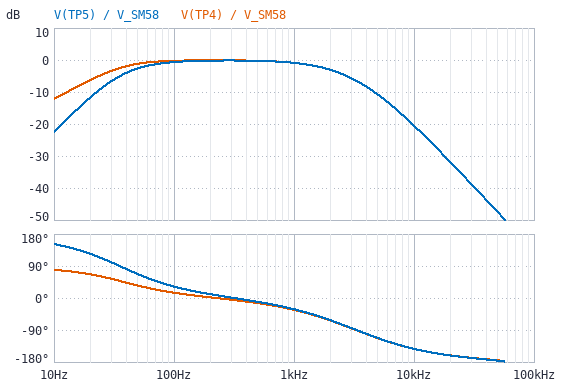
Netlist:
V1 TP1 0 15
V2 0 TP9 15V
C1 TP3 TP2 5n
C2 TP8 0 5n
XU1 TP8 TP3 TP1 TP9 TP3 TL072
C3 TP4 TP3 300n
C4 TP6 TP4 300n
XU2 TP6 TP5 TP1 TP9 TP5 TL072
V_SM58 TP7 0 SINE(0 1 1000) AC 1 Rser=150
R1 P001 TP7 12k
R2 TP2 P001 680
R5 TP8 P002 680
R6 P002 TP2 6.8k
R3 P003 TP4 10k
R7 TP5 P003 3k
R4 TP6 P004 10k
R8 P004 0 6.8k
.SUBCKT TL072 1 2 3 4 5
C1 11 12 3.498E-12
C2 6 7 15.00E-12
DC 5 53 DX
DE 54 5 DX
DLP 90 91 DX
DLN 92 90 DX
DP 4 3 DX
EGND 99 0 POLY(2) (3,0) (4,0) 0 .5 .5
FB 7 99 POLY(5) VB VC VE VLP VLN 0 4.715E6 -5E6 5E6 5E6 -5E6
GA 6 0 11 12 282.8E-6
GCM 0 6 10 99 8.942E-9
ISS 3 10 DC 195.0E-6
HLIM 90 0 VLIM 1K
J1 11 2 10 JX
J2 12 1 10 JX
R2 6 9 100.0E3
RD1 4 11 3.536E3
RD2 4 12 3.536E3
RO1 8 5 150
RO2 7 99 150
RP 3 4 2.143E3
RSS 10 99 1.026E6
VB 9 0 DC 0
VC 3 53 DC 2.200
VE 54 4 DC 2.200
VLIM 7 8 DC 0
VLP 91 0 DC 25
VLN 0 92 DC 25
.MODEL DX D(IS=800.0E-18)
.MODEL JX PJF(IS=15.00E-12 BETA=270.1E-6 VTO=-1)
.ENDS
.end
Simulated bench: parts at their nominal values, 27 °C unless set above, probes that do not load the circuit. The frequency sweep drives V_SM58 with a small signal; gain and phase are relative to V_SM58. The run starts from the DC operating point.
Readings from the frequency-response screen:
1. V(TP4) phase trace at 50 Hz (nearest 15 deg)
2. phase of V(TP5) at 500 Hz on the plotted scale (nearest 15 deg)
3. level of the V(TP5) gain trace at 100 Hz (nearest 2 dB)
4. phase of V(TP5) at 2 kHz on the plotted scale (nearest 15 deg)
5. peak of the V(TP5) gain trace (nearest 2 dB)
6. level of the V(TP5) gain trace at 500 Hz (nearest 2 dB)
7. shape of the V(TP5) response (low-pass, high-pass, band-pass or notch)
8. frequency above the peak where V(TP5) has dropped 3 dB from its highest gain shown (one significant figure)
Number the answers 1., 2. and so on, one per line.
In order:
1. 30 deg
2. -15 deg
3. 0 dB
4. -60 deg
5. 0 dB
6. 0 dB
7. band-pass
8. 2 kHz
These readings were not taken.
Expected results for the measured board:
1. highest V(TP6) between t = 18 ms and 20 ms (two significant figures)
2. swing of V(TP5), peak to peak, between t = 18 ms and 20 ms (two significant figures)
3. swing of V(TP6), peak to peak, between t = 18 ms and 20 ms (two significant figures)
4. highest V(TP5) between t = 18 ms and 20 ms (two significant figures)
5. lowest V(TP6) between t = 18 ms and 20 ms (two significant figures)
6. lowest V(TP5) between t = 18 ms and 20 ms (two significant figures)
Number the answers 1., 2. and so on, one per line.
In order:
1. 900 mV
2. 1.8 V
3. 1.8 V
4. 900 mV
5. -900 mV
6. -900 mV
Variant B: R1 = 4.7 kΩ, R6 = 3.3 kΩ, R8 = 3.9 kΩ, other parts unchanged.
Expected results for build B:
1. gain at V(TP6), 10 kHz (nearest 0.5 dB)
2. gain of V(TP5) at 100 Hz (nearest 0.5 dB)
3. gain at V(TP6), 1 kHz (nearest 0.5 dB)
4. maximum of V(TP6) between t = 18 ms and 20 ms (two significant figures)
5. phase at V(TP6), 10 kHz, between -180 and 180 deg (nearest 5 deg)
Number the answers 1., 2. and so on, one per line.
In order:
1. -10.0 dB
2. -1.0 dB
3. 0 dB
4. 980 mV
5. -110 deg
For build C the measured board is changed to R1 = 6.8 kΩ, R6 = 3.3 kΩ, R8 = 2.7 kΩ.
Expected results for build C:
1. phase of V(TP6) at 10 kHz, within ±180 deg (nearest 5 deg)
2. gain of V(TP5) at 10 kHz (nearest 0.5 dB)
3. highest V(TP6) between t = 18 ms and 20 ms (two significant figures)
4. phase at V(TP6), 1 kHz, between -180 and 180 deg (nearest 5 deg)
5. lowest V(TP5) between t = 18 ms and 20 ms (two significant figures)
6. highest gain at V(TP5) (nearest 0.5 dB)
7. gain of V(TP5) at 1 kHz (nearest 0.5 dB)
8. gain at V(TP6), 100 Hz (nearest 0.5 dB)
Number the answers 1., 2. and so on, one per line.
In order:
1. -120 deg
2. -12.5 dB
3. 960 mV
4. -15 deg
5. -960 mV
6. 0 dB
7. -0.5 dB
8. -1.5 dB
